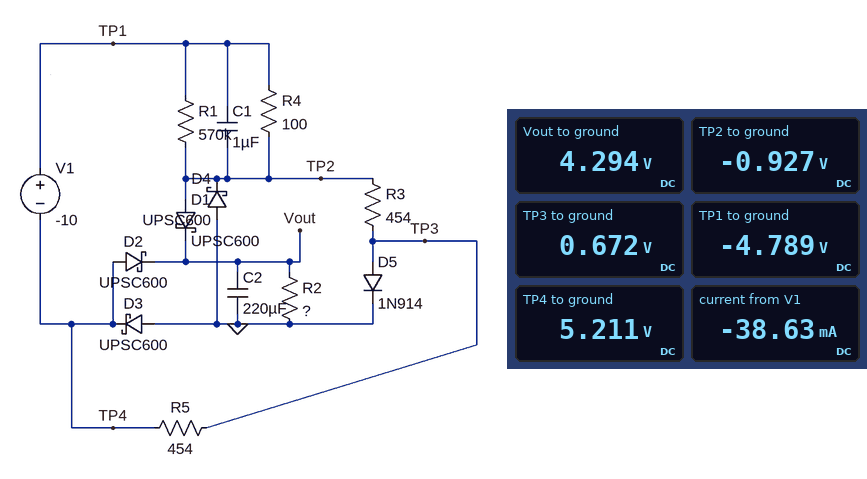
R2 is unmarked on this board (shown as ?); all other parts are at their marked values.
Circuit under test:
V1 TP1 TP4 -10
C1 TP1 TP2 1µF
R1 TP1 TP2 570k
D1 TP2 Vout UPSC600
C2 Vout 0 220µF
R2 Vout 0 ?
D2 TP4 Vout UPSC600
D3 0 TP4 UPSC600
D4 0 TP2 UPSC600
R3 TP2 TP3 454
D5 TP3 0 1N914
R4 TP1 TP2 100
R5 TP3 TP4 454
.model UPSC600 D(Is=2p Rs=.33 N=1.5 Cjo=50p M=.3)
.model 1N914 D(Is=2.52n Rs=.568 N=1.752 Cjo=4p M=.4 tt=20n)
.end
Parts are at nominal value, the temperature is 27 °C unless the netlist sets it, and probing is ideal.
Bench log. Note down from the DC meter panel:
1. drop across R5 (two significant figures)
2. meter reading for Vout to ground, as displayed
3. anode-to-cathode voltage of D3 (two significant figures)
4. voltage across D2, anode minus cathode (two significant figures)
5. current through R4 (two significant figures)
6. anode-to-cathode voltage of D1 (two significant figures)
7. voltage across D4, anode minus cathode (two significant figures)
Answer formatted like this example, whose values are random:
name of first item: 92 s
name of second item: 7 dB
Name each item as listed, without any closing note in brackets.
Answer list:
drop across R5: 4.5 V
meter reading for Vout to ground, as displayed: 4.294 V
anode-to-cathode voltage of D3: -5.2 V
voltage across D2, anode minus cathode: 920 mV
current through R4: 39 mA
anode-to-cathode voltage of D1: -5.2 V
voltage across D4, anode minus cathode: 930 mV
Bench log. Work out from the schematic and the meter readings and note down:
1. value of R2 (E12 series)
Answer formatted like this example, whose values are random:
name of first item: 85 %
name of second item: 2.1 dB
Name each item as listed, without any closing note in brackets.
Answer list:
value of R2: 150 Ω
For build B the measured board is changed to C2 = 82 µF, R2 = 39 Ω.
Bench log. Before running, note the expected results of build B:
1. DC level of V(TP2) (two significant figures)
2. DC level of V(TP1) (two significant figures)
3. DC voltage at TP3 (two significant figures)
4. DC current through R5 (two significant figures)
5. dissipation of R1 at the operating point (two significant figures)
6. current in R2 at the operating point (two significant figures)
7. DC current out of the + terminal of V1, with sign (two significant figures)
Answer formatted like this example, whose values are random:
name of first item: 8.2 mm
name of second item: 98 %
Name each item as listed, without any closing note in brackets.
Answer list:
DC level of V(TP2): -950 mV
DC level of V(TP1): -6.9 V
DC voltage at TP3: 620 mV
DC current through R5: 5.4 mA
dissipation of R1 at the operating point: 63 µW
current in R2 at the operating point: 54 mA
DC current out of the + terminal of V1, with sign: -60 mA
